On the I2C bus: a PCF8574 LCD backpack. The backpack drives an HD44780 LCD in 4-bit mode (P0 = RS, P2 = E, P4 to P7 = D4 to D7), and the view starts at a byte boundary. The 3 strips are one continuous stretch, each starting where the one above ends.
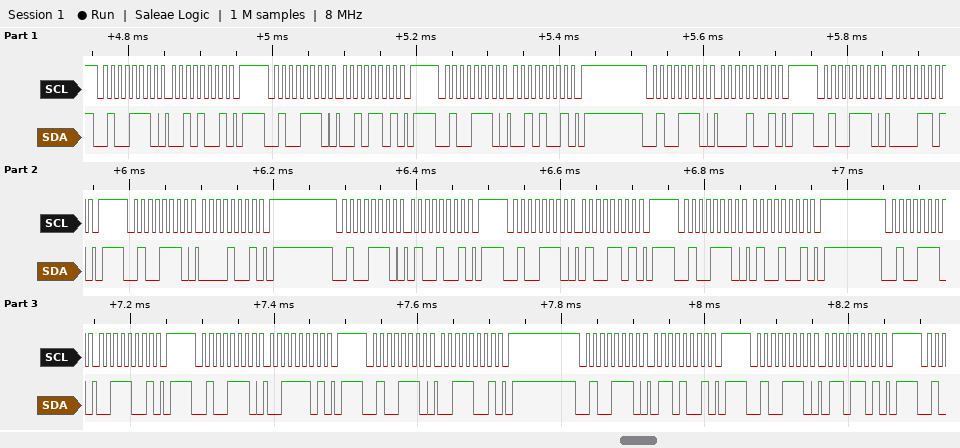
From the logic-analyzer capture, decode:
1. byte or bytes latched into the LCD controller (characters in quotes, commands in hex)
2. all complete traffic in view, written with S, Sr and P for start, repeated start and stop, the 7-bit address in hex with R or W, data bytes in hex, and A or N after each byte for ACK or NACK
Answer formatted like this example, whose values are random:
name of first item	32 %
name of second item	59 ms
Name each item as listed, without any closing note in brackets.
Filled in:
byte or bytes latched into the LCD controller	' ' 'C'
all complete traffic in view, written with S, Sr and P for start, repeated start and stop, the 7-bit address in hex with R or W, data bytes in hex, and A or N after each byte for ACK or NACK	S 27W A 29 A P S 27W A 2D A P S 27W A 29 A P S 27W A 09 A P S 27W A 0D A P S 27W A 09 A P S 27W A 49 A P S 27W A 4D A P S 27W A 49 A P S 27W A 39 A P S 27W A 3D A P S 27W A 39 A P S 27W A 69 A P S 27W A 6D A P
